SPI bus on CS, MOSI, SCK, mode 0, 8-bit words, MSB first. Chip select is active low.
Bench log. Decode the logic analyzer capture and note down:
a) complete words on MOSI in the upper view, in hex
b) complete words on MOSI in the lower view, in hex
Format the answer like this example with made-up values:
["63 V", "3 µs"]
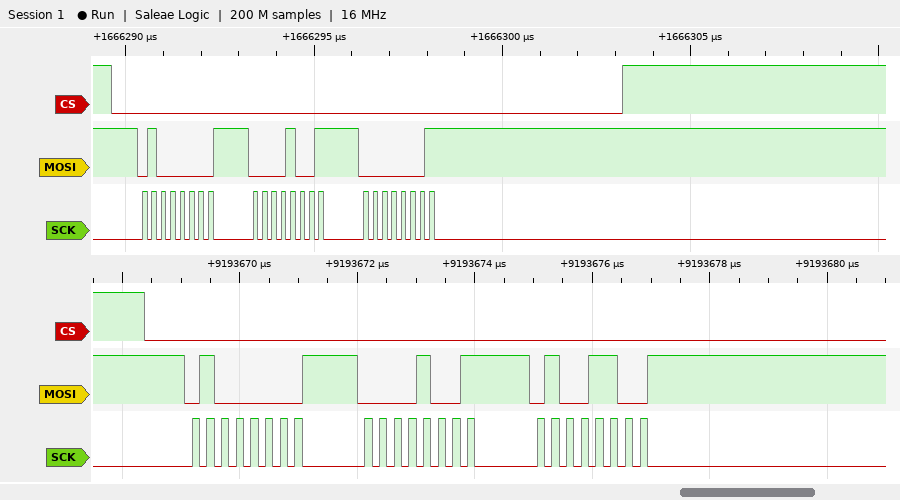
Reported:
["40, 09, 01", "40, 09, 4C"]
